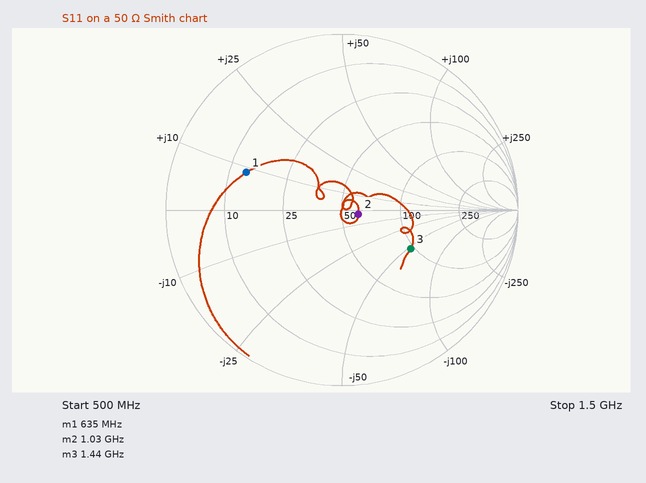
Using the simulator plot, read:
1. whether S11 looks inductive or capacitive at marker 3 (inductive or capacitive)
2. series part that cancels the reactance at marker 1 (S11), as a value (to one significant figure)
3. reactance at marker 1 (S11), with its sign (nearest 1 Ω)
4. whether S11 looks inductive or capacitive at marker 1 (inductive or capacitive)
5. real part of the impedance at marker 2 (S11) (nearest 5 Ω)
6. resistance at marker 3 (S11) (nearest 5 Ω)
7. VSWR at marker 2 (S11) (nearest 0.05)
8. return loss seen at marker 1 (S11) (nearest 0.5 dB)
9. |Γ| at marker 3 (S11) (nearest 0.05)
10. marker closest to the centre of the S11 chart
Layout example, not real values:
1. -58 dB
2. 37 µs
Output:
1. capacitive
2. 30 pF
3. +9 Ω
4. inductive
5. 60 Ω
6. 95 Ω
7. 1.20
8. 4.5 dB
9. 0.45
10. marker 2
